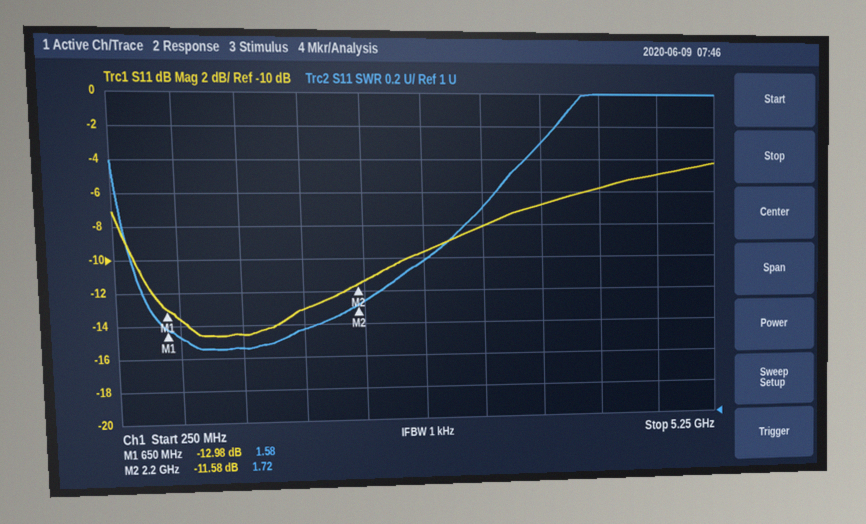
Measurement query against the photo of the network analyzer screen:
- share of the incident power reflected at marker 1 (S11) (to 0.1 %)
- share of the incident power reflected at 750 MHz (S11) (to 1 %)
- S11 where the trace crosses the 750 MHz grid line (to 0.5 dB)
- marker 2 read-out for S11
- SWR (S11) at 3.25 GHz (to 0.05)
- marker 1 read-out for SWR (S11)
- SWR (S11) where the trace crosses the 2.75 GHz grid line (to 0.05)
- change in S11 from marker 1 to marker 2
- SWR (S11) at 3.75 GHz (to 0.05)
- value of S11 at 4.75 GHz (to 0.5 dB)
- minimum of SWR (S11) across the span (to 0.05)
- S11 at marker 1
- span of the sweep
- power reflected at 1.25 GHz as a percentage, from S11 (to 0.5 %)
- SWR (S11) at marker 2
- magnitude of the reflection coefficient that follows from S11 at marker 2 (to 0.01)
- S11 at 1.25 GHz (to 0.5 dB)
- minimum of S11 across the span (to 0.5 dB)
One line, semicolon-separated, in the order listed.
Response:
5.0 %; 4 %; -13.5 dB; -11.58 dB; 2.30; 1.58; 2.00; 1.40 dB; 2.70; -5.0 dB; 1.45; -12.98 dB; 5 GHz; 3.5 %; 1.72; 0.26; -14.5 dB; -14.5 dB
